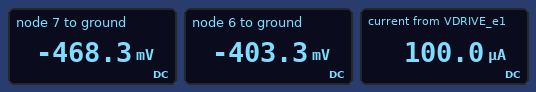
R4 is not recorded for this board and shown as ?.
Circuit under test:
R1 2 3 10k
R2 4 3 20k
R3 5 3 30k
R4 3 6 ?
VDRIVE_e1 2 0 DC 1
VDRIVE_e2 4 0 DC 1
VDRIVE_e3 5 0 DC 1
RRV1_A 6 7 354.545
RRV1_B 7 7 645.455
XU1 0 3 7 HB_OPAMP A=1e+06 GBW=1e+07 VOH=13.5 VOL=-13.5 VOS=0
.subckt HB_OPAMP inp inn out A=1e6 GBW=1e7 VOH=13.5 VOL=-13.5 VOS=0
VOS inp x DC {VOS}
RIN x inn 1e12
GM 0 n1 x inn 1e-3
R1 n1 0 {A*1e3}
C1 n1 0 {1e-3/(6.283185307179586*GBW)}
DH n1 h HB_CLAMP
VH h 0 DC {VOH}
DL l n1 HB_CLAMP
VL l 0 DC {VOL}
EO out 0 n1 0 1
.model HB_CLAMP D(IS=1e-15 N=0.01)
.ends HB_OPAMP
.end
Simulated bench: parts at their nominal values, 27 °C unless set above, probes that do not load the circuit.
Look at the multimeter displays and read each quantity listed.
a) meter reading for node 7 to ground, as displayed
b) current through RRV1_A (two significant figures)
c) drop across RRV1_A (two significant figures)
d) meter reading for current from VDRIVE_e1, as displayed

-468.3 mV
180 µA
65 mV
100.0 µA
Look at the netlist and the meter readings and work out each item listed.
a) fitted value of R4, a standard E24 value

2.2 kΩ
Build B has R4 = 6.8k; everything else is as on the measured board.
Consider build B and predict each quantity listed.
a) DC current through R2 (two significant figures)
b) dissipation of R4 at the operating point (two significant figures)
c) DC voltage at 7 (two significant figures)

50 µA
230 µW
-1.3 V
